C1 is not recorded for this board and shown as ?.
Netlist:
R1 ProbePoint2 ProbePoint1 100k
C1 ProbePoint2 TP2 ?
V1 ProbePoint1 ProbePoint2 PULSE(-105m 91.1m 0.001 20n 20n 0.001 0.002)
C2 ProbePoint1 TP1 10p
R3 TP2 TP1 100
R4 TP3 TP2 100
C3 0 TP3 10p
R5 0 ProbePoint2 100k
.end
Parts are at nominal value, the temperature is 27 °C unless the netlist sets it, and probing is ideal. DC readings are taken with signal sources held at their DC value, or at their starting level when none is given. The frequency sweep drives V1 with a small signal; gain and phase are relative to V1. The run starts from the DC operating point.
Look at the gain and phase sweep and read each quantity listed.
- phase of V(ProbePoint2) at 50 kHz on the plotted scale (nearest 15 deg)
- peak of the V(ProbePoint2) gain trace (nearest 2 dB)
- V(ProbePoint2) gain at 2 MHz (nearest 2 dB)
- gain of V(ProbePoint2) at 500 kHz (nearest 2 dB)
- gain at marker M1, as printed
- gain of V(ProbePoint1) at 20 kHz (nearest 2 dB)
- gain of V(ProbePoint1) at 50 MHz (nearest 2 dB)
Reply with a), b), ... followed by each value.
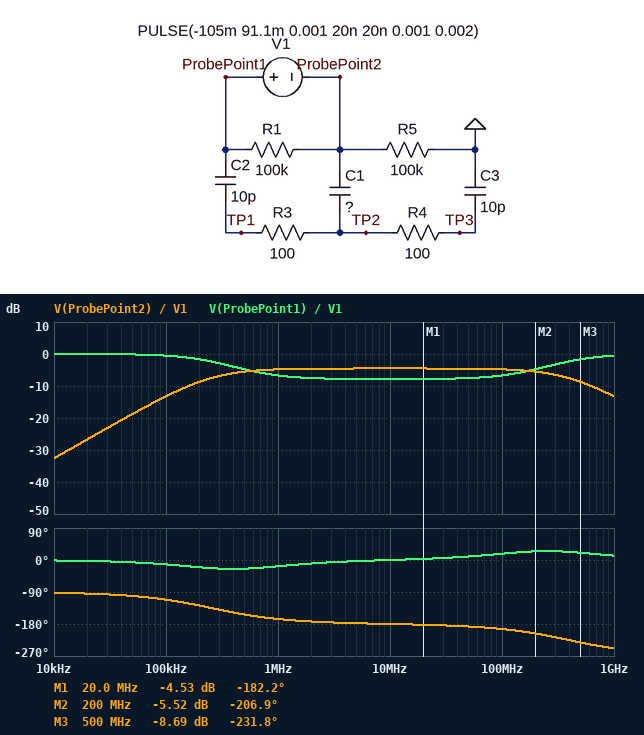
a) -105 deg
b) -4 dB
c) -4 dB
d) -6 dB
e) -4.53 dB
f) 0 dB
g) -8 dB
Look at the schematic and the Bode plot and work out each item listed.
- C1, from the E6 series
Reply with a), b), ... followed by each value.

a) 6.8 pF
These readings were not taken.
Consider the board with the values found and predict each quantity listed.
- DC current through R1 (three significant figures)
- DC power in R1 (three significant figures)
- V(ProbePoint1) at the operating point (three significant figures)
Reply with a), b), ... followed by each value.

a) 1.05 µA
b) 110 nW
c) -105 mV
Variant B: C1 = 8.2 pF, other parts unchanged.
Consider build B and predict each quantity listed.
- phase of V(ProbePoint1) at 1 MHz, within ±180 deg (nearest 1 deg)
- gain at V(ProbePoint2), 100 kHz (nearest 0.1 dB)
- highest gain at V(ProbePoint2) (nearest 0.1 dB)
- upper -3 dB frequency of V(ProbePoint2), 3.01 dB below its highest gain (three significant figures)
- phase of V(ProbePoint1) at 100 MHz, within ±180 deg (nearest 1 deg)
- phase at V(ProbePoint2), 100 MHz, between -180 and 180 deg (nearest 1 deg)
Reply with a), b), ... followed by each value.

a) -15 deg
b) -13.7 dB
c) -5.2 dB
d) 354 MHz
e) 16 deg
f) 164 deg
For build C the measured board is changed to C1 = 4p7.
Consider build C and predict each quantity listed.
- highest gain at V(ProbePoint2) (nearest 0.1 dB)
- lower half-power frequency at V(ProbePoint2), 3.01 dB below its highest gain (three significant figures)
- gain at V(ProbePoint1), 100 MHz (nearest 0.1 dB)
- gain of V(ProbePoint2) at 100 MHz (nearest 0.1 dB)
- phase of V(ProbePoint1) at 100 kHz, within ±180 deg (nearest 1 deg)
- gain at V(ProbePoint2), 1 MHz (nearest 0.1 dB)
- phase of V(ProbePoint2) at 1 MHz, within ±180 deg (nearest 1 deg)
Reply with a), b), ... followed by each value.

a) -3.4 dB
b) 267 kHz
c) -8.6 dB
d) -3.5 dB
e) -14 deg
f) -3.7 dB
g) -165 deg
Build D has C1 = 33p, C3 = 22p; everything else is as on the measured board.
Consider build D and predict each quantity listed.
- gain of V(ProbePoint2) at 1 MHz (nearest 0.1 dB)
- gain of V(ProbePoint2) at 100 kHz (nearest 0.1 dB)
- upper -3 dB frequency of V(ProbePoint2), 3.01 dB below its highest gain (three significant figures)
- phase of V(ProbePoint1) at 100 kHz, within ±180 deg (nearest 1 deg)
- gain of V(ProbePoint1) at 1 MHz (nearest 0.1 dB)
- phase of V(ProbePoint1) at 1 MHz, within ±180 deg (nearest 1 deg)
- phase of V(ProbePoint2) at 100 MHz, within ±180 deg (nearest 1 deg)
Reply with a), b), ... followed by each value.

a) -12.7 dB
b) -16.1 dB
c) 208 MHz
d) -7 deg
e) -2.3 dB
f) -2 deg
g) 154 deg
